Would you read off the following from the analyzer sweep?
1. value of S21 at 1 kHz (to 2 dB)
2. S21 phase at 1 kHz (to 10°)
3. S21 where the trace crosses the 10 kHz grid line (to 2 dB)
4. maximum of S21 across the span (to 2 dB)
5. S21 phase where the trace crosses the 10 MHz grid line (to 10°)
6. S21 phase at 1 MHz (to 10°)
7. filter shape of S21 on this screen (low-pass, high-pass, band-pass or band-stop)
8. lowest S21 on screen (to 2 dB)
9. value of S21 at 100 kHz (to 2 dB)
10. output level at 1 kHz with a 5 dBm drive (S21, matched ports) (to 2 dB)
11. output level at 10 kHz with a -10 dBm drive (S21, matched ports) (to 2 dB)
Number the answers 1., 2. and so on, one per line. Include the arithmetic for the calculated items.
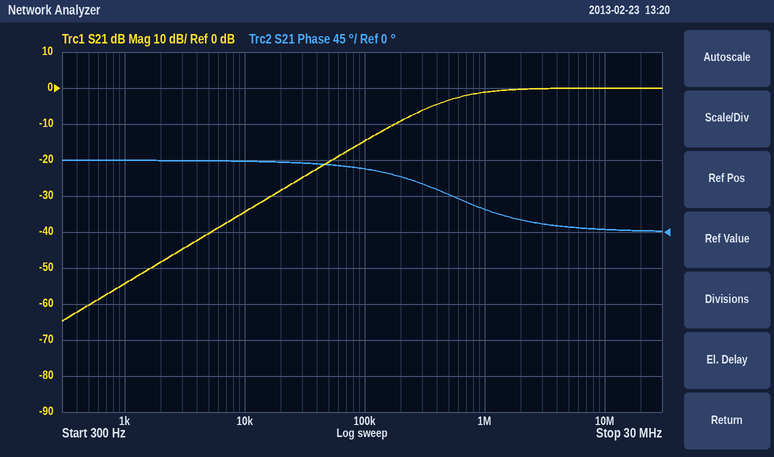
1. -54 dB
2. 90°
3. -34 dB
4. 0 dB
5. 0°
6. 30°
7. high-pass
8. -64 dB
9. -14 dB
10. 5 dBm + (-54 dB) = -50 dBm
11. -10 dBm + (-34 dB) = -44 dBm
